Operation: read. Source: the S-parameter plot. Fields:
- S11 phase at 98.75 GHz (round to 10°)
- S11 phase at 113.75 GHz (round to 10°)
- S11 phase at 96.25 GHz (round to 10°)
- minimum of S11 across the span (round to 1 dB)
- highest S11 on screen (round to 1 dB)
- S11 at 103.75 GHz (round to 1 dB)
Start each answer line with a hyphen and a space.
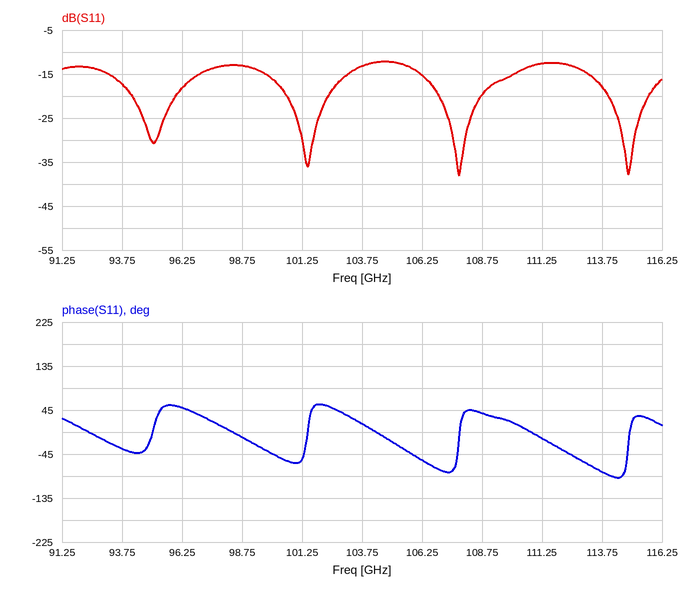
- -10°
- -80°
- 50°
- -38 dB
- -12 dB
- -13 dB
